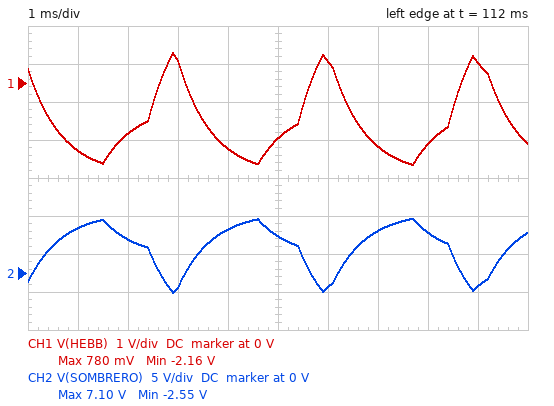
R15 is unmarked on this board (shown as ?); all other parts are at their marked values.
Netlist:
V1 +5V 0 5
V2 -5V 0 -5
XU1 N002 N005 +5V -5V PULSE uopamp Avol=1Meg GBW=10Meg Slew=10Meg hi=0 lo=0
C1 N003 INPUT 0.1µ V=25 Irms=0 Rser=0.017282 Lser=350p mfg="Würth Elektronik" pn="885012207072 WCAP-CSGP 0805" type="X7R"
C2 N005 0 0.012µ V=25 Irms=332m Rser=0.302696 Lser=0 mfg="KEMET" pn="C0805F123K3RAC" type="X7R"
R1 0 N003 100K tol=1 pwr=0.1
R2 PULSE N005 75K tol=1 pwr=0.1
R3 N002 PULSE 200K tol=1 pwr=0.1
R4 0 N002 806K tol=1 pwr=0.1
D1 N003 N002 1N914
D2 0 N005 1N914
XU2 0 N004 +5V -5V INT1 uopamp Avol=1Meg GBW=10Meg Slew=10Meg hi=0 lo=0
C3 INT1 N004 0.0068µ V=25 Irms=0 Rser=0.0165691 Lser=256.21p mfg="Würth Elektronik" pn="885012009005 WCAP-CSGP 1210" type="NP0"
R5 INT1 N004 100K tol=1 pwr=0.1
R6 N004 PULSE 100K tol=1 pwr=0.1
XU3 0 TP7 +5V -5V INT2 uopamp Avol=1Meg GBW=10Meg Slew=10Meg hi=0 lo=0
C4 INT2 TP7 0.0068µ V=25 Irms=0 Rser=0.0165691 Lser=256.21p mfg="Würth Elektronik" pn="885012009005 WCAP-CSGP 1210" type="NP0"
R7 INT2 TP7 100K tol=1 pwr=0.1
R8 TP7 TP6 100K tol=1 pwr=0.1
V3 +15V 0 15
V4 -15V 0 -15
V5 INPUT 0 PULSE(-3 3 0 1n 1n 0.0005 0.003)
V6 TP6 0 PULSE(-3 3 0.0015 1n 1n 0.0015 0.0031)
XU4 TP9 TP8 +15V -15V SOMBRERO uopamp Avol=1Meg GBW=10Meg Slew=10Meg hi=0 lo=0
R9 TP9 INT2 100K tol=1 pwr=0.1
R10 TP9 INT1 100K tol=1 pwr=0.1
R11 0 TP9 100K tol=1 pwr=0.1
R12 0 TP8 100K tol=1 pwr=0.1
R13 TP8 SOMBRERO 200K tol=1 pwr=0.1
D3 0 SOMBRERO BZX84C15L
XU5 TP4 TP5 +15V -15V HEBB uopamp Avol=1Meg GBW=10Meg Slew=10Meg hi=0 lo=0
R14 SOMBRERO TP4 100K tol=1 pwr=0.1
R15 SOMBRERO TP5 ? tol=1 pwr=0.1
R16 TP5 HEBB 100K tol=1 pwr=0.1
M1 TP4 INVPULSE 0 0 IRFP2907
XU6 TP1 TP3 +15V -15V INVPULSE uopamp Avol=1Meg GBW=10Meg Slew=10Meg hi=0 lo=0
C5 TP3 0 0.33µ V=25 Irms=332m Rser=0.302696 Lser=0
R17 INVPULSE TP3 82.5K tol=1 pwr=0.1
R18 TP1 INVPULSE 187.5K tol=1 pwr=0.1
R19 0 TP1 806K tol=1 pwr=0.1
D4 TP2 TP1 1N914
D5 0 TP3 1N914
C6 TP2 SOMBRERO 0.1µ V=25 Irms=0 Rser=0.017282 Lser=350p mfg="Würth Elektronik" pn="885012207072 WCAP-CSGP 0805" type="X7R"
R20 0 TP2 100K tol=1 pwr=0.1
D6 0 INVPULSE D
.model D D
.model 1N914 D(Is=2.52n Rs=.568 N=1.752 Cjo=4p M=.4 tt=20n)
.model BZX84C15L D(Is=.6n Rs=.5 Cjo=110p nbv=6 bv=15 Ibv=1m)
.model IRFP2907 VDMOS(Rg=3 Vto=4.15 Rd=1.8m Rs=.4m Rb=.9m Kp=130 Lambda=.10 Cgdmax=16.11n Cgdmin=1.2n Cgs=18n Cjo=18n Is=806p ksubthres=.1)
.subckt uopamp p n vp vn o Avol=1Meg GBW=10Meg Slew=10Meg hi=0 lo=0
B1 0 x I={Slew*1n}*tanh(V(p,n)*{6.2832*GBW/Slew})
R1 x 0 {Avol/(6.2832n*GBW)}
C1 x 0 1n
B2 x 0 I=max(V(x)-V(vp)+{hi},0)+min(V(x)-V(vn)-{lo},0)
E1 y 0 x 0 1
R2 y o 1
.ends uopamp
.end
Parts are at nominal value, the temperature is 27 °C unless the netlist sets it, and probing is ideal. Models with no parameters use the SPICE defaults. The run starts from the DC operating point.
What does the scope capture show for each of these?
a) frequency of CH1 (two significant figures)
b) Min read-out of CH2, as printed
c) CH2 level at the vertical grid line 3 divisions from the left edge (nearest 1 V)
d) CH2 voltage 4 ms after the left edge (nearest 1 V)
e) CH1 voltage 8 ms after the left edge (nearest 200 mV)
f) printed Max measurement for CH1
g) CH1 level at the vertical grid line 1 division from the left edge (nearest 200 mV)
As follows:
330 Hz
-2.55 V
-2 V
6 V
-1.6 V
780 mV
-1.8 V
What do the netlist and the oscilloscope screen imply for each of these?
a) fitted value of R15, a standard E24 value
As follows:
330 kΩ
